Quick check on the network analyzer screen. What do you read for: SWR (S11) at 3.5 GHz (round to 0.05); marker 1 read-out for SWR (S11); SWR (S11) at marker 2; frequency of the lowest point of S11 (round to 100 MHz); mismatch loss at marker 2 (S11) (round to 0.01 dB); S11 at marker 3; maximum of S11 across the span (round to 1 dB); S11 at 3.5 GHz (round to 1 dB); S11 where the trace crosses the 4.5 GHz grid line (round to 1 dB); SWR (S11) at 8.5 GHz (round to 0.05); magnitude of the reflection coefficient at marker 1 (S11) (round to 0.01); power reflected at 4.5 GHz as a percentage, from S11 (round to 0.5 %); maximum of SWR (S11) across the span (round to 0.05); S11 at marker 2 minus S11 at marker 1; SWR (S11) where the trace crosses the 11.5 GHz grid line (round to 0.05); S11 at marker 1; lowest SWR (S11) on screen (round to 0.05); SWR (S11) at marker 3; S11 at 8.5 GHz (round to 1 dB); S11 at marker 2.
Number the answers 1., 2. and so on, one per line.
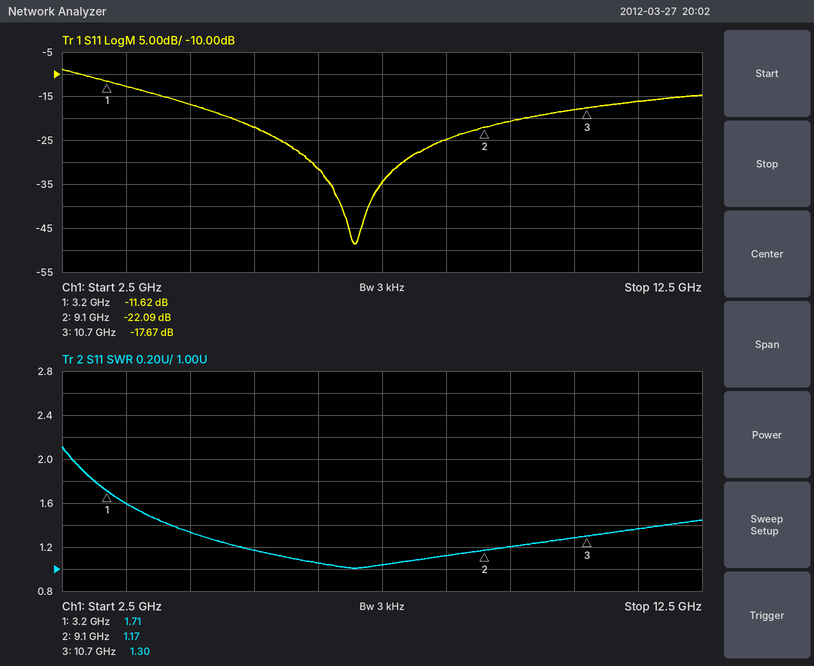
1. 1.60
2. 1.71
3. 1.17
4. 7.1 GHz
5. 0.03 dB
6. -17.67 dB
7. -9 dB
8. -13 dB
9. -17 dB
10. 1.10
11. 0.26
12. 2.0 %
13. 2.10
14. -10.47 dB
15. 1.35
16. -11.62 dB
17. 1.00
18. 1.30
19. -25 dB
20. -22.09 dB
